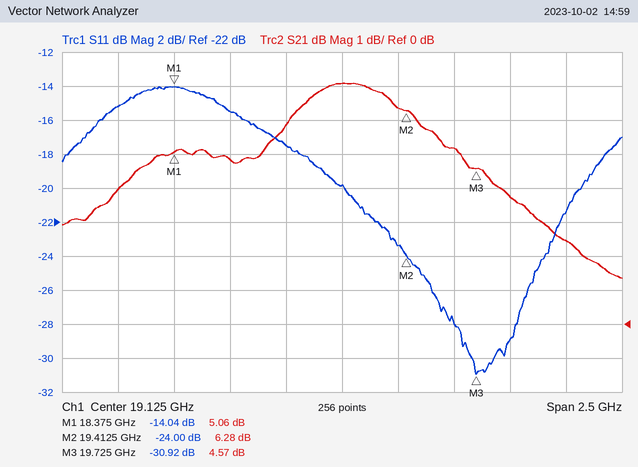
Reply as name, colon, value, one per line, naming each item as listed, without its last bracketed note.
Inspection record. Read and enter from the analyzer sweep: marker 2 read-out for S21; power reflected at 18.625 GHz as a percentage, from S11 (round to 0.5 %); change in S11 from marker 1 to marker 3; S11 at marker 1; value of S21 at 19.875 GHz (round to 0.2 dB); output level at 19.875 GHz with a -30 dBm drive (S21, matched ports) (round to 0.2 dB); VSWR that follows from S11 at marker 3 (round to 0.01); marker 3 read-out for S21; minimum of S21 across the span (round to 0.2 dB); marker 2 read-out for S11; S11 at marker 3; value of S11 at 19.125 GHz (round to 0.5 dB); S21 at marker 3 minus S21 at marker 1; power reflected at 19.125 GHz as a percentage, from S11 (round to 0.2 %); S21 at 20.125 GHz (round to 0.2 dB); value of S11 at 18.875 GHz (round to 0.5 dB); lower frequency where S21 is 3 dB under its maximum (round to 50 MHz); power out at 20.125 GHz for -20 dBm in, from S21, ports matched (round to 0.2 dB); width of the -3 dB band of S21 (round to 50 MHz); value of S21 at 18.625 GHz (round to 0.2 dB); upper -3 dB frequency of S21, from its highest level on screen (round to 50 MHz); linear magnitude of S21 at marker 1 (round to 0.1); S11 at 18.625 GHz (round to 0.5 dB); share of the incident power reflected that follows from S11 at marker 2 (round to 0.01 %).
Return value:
marker 2 read-out for S21: 6.28 dB
power reflected at 18.625 GHz as a percentage, from S11: 3.0 %
change in S11 from marker 1 to marker 3: -16.88 dB
S11 at marker 1: -14.04 dB
value of S21 at 19.875 GHz: 3.8 dB
output level at 19.875 GHz with a -30 dBm drive (S21, matched ports): -26.2 dBm
VSWR that follows from S11 at marker 3: 1.06
marker 3 read-out for S21: 4.57 dB
minimum of S21 across the span: 1.4 dB
marker 2 read-out for S11: -24.00 dB
S11 at marker 3: -30.92 dB
value of S11 at 19.125 GHz: -20.0 dB
S21 at marker 3 minus S21 at marker 1: -0.49 dB
power reflected at 19.125 GHz as a percentage, from S11: 1.0 %
S21 at 20.125 GHz: 2.4 dB
value of S11 at 18.875 GHz: -17.5 dB
lower frequency where S21 is 3 dB under its maximum: 18.15 GHz
power out at 20.125 GHz for -20 dBm in, from S21, ports matched: -17.6 dBm
width of the -3 dB band of S21: 1.65 GHz
value of S21 at 18.625 GHz: 4.8 dB
upper -3 dB frequency of S21, from its highest level on screen: 19.80 GHz
linear magnitude of S21 at marker 1: 1.8
S11 at 18.625 GHz: -15.5 dB
share of the incident power reflected that follows from S11 at marker 2: 0.40 %
